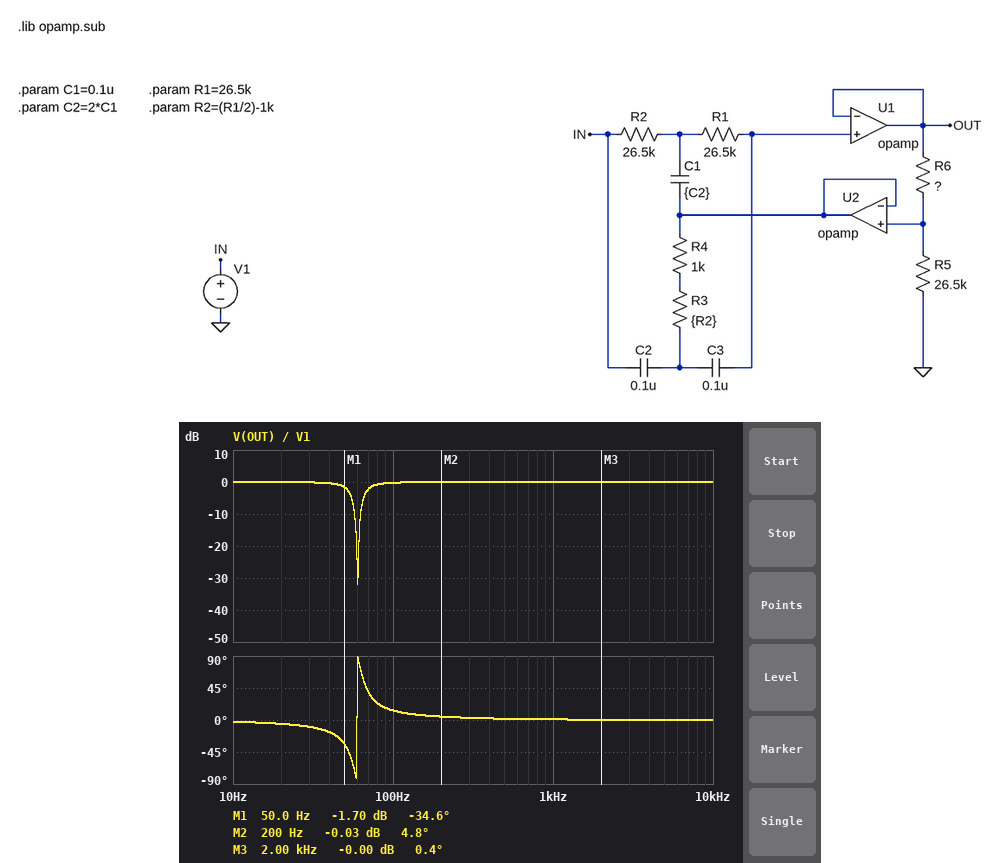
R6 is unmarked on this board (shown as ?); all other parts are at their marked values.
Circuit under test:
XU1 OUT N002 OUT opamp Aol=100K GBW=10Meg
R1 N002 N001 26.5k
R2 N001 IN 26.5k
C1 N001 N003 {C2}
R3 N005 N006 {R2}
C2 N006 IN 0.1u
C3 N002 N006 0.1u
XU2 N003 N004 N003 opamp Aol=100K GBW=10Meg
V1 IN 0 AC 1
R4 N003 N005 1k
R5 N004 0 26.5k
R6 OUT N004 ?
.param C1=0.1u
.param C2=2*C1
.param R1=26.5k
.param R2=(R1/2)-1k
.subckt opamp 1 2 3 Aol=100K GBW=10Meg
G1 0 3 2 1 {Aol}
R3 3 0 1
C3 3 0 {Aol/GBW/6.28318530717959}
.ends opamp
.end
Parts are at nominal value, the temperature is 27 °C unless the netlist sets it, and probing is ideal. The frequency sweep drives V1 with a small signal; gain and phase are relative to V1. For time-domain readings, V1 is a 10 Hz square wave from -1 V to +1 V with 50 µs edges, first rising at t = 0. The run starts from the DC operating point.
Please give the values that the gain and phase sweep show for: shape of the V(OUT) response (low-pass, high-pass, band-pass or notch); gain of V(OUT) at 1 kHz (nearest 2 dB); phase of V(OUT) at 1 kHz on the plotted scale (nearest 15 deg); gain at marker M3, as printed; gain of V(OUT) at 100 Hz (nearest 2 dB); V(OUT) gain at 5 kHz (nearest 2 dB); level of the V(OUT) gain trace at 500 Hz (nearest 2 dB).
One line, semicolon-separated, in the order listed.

notch; 0 dB; 0 deg; -0.00 dB; 0 dB; 0 dB; 0 dB
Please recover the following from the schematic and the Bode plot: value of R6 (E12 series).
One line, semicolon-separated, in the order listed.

1.8 kΩ
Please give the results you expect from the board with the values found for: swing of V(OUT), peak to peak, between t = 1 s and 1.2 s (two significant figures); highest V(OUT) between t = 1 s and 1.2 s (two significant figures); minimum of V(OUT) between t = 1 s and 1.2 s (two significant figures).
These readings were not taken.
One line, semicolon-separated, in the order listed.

2.5 V; 1.3 V; -1.3 V
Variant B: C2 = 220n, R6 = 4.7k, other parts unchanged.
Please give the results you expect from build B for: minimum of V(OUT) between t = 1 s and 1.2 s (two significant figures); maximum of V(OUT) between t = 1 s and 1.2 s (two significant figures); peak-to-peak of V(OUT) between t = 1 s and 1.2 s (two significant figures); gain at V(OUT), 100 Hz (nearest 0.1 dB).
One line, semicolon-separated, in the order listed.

-1.2 V; 1.2 V; 2.3 V; -0.6 dB
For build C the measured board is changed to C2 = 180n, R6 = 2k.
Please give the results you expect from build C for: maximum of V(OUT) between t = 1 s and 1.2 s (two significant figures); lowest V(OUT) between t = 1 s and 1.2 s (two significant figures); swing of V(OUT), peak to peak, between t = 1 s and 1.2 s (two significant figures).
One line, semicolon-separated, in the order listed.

1.2 V; -1.2 V; 2.4 V
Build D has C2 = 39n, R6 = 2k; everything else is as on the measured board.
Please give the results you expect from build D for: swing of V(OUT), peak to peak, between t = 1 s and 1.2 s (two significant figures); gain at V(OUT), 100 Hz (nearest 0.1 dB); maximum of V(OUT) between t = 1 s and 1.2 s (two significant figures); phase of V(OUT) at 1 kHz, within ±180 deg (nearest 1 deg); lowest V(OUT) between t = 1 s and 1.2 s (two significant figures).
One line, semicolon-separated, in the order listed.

2.9 V; -1.4 dB; 1.5 V; 2 deg; -1.5 V
